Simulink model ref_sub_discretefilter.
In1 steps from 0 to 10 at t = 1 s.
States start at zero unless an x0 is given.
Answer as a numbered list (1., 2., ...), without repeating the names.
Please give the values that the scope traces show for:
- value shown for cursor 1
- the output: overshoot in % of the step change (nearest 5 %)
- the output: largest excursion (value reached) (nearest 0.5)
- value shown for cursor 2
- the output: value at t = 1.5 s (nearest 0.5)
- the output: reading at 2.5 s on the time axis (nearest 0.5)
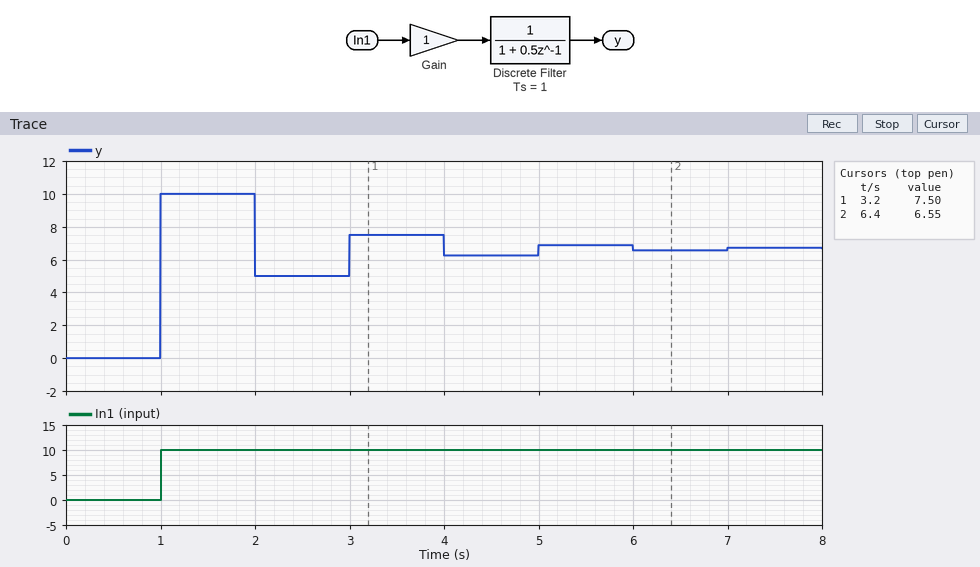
1. 7.50
2. 50 %
3. 10.0
4. 6.55
5. 10.0
6. 5.0
